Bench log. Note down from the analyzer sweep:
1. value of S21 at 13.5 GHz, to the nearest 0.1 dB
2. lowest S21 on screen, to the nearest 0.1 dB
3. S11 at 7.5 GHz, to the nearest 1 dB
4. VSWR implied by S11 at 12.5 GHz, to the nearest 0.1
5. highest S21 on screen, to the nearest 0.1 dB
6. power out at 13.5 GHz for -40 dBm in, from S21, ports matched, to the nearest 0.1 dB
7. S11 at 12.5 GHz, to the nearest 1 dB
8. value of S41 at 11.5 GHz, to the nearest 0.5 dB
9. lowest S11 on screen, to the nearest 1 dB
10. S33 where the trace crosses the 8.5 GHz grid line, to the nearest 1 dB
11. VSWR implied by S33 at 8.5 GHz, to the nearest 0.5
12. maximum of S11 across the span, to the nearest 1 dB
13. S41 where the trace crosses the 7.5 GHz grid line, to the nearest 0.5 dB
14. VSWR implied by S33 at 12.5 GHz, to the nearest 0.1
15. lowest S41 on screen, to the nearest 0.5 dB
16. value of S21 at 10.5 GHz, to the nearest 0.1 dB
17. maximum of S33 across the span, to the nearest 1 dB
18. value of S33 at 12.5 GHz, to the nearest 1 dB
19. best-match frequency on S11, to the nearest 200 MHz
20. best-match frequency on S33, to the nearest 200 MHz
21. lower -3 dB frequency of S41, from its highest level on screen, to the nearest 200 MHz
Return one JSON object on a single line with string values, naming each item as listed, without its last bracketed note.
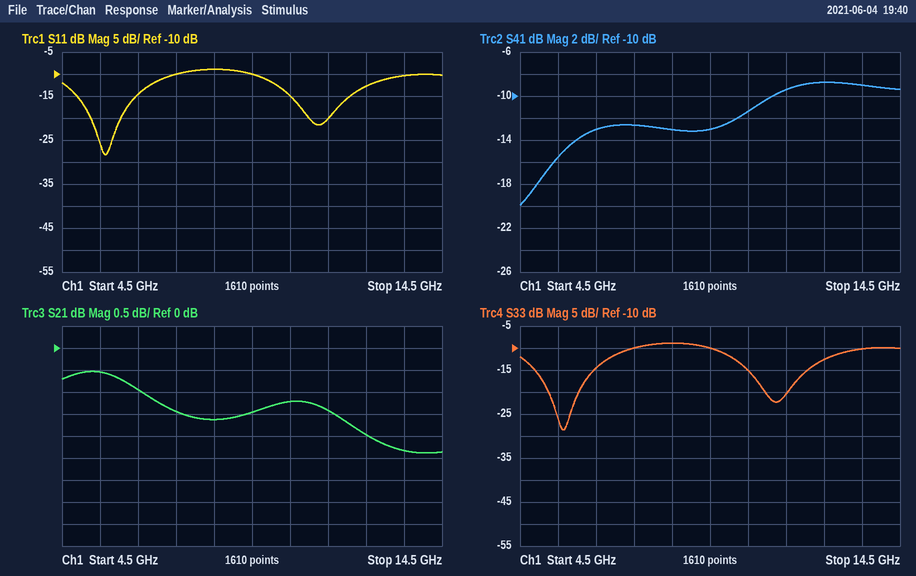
{"value of S21 at 13.5 GHz, to the nearest 0.1 dB": "-2.3 dB", "lowest S21 on screen, to the nearest 0.1 dB": "-2.4 dB", "S11 at 7.5 GHz, to the nearest 1 dB": "-10 dB", "VSWR implied by S11 at 12.5 GHz, to the nearest 0.1": "1.6", "highest S21 on screen, to the nearest 0.1 dB": "-0.5 dB", "power out at 13.5 GHz for -40 dBm in, from S21, ports matched, to the nearest 0.1 dB": "-42.3 dBm", "S11 at 12.5 GHz, to the nearest 1 dB": "-13 dB", "value of S41 at 11.5 GHz, to the nearest 0.5 dB": "-9.5 dB", "lowest S11 on screen, to the nearest 1 dB": "-28 dB", "S33 where the trace crosses the 8.5 GHz grid line, to the nearest 1 dB": "-9 dB", "VSWR implied by S33 at 8.5 GHz, to the nearest 0.5": "2.0", "maximum of S11 across the span, to the nearest 1 dB": "-9 dB", "S41 where the trace crosses the 7.5 GHz grid line, to the nearest 0.5 dB": "-12.5 dB", "VSWR implied by S33 at 12.5 GHz, to the nearest 0.1": "1.6", "lowest S41 on screen, to the nearest 0.5 dB": "-20.0 dB", "value of S21 at 10.5 GHz, to the nearest 0.1 dB": "-1.2 dB", "maximum of S33 across the span, to the nearest 1 dB": "-9 dB", "value of S33 at 12.5 GHz, to the nearest 1 dB": "-13 dB", "best-match frequency on S11, to the nearest 200 MHz": "5.6 GHz", "best-match frequency on S33, to the nearest 200 MHz": "5.6 GHz", "lower -3 dB frequency of S41, from its highest level on screen, to the nearest 200 MHz": "10.4 GHz"}
